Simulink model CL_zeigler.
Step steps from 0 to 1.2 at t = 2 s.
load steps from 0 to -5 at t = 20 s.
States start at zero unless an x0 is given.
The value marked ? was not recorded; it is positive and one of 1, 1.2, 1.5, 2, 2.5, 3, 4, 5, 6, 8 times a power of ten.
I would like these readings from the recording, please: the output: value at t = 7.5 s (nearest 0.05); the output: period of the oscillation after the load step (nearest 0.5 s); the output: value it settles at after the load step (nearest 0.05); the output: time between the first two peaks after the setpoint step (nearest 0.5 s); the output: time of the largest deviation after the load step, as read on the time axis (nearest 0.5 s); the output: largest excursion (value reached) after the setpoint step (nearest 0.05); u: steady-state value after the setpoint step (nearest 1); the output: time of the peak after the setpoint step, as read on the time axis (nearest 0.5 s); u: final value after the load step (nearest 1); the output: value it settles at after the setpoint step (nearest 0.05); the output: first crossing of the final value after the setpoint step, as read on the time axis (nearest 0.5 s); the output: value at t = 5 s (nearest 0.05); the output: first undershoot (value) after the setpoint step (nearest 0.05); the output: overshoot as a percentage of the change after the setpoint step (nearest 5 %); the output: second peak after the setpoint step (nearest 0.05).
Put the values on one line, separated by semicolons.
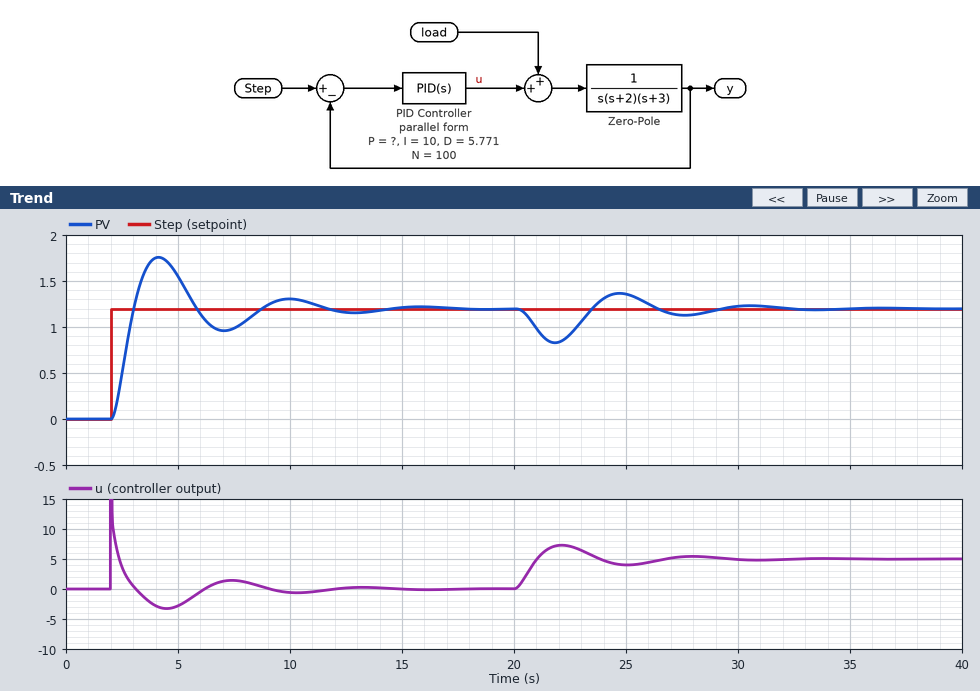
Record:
1.00; 6.0 s; 1.20; 6.0 s; 22.0 s; 1.75; 0; 4.0 s; 5; 1.20; 3.0 s; 1.55; 0.95; 45 %; 1.30
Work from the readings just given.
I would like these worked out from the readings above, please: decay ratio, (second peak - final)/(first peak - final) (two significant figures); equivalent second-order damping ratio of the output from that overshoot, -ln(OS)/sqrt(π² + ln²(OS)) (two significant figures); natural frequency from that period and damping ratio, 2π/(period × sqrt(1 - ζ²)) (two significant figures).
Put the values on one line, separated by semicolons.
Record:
0.18; 0.25; 1.1 rad/s
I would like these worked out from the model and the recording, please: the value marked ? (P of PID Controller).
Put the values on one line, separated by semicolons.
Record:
10
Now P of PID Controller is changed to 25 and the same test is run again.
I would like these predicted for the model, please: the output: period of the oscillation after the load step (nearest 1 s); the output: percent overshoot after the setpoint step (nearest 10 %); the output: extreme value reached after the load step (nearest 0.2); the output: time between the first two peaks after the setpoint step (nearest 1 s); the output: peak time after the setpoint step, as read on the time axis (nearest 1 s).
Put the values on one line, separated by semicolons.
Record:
3 s; 60 %; 1.0; 3 s; 3 s
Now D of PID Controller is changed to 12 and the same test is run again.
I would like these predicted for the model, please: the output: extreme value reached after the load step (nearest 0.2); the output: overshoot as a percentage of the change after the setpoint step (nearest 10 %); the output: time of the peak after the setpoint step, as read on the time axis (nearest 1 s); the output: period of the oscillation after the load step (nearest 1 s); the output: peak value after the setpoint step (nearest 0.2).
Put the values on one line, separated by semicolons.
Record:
1.0; 20 %; 5 s; 8 s; 1.4
